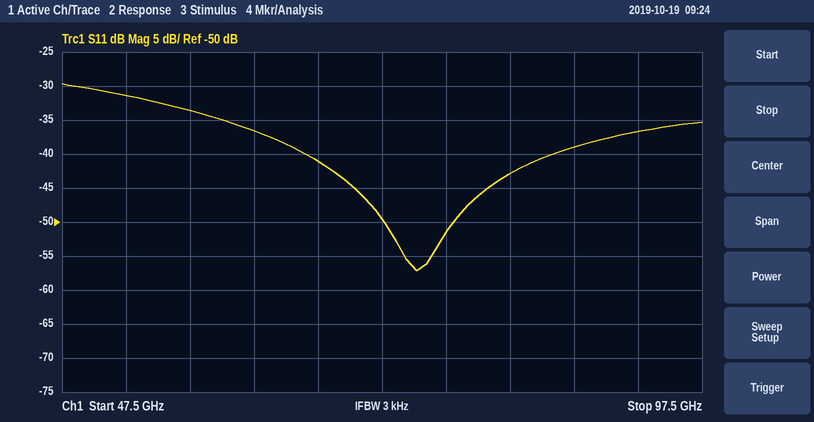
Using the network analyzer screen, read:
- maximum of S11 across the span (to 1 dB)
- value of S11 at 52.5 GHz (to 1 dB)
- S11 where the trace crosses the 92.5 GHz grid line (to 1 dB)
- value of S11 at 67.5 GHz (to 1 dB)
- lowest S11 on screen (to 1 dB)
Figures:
-30 dB
-31 dB
-37 dB
-41 dB
-57 dB
